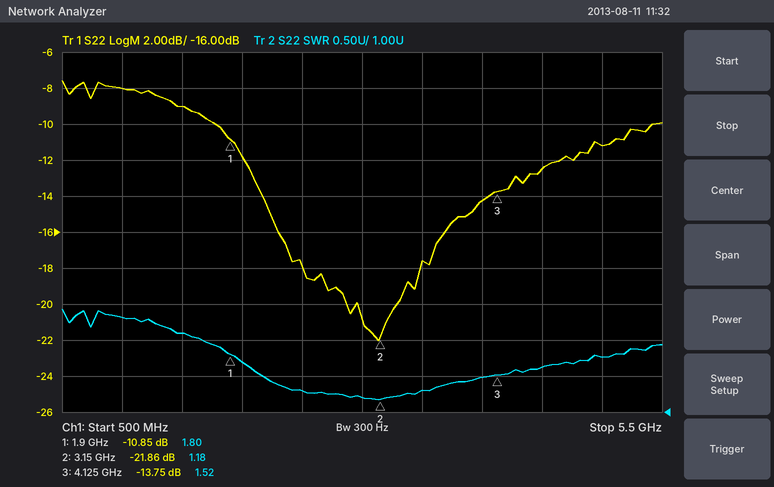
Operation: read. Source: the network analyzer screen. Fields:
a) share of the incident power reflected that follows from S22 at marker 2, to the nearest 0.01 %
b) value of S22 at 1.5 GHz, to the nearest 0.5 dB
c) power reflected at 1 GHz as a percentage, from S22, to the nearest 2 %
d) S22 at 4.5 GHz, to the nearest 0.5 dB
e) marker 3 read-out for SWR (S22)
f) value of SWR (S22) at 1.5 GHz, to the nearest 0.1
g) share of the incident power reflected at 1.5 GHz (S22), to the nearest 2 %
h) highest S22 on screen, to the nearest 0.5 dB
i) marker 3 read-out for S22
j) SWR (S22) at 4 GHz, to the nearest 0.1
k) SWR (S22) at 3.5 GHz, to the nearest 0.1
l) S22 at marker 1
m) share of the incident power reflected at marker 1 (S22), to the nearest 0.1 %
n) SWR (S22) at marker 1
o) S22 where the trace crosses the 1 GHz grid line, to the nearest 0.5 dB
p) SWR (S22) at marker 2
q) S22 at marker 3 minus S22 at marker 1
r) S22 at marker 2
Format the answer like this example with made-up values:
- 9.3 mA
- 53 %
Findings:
- 0.65 %
- -9.0 dB
- 16 %
- -12.5 dB
- 1.52
- 2.1
- 12 %
- -7.5 dB
- -13.75 dB
- 1.5
- 1.3
- -10.85 dB
- 8.2 %
- 1.80
- -8.0 dB
- 1.18
- -2.90 dB
- -21.86 dB
